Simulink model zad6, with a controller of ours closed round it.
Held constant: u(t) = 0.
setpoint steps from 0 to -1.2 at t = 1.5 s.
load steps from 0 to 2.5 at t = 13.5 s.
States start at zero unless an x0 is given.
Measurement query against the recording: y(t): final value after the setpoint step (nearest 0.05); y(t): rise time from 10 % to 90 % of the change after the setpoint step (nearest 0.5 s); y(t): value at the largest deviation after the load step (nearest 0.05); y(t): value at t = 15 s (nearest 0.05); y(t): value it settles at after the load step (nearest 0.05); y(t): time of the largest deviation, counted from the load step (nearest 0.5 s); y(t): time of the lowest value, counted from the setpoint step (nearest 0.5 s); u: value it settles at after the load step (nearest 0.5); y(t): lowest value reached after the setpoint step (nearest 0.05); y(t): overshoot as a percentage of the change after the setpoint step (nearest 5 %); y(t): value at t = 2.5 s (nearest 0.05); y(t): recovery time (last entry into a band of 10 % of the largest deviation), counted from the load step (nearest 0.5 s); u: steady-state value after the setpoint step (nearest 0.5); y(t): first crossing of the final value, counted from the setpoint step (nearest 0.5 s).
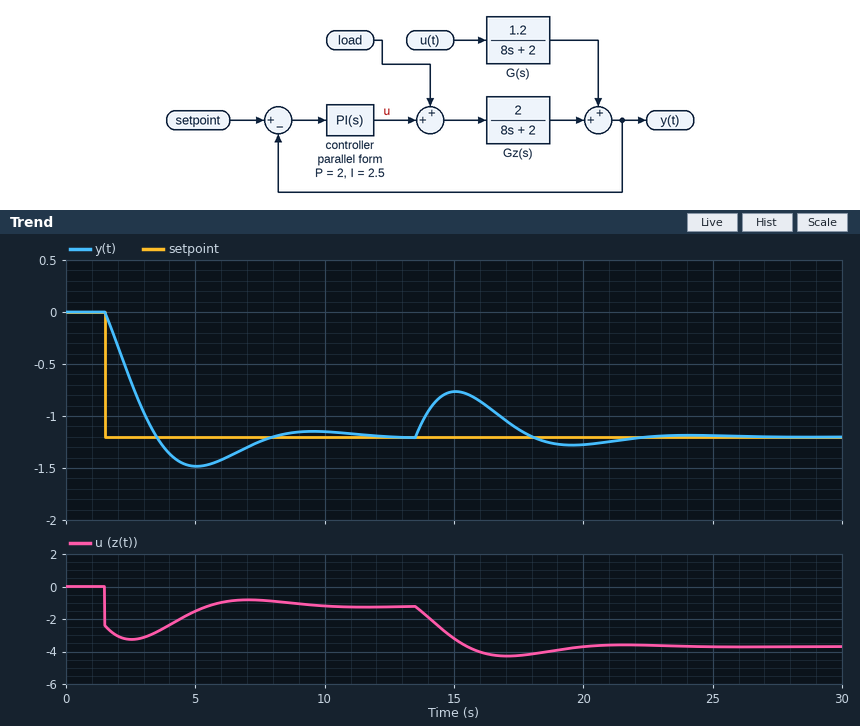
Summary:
-1.20
1.5 s
-0.75
-0.75
-1.20
1.5 s
3.5 s
-3.5
-1.50
25 %
-0.65
7.5 s
-1.0
2.0 s
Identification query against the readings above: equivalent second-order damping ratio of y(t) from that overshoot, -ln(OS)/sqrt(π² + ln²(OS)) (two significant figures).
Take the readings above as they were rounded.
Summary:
0.40
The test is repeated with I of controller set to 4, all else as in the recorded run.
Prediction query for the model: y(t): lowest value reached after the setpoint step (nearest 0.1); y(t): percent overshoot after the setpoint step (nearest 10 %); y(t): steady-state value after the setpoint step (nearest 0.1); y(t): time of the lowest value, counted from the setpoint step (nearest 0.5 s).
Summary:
-1.6
30 %
-1.2
3.0 s
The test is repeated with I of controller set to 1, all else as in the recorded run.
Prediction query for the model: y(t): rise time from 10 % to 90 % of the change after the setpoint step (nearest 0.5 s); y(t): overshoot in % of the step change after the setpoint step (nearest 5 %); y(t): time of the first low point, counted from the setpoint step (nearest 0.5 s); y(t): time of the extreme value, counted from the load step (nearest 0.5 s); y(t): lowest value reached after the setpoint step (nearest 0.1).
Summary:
2.5 s
10 %
6.0 s
2.0 s
-1.3
